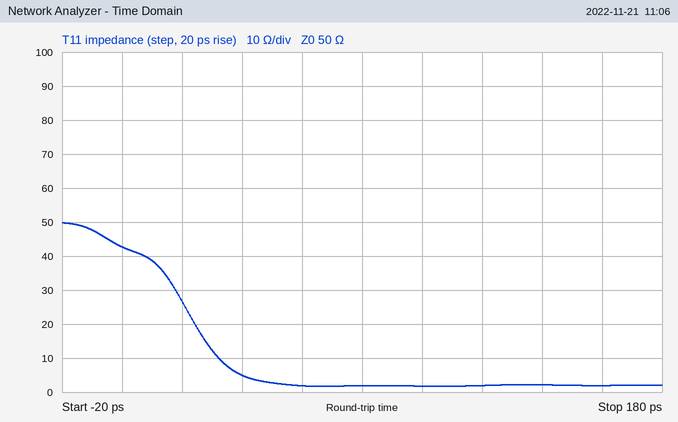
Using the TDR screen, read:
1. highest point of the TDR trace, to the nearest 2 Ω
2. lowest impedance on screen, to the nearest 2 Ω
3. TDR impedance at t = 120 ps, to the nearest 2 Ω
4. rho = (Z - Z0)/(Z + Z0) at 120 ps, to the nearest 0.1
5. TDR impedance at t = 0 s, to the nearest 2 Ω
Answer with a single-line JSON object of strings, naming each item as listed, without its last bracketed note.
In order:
{"highest point of the TDR trace, to the nearest 2 Ω": "50 Ω", "lowest impedance on screen, to the nearest 2 Ω": "2 Ω", "TDR impedance at t = 120 ps, to the nearest 2 Ω": "2 Ω", "rho = (Z - Z0)/(Z + Z0) at 120 ps, to the nearest 0.1": "-0.9", "TDR impedance at t = 0 s, to the nearest 2 Ω": "42 Ω"}
